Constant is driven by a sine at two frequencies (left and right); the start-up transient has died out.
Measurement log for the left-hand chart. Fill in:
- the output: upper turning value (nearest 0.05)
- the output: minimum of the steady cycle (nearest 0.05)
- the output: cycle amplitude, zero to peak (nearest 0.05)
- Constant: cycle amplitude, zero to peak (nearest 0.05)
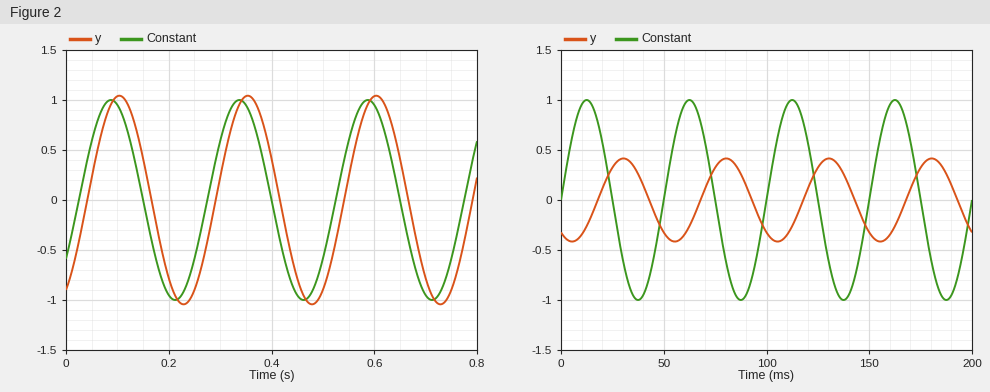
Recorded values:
1.05
-1.05
1.05
1.00
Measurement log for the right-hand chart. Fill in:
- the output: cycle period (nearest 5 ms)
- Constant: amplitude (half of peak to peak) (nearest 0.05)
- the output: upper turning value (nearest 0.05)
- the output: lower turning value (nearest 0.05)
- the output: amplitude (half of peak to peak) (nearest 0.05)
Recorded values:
50 ms
1.00
0.40
-0.40
0.40
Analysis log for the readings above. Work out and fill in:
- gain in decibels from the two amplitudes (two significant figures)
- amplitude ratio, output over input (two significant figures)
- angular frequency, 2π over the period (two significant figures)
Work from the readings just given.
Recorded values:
-8.0 dB
0.40
0.13 rad/ms
